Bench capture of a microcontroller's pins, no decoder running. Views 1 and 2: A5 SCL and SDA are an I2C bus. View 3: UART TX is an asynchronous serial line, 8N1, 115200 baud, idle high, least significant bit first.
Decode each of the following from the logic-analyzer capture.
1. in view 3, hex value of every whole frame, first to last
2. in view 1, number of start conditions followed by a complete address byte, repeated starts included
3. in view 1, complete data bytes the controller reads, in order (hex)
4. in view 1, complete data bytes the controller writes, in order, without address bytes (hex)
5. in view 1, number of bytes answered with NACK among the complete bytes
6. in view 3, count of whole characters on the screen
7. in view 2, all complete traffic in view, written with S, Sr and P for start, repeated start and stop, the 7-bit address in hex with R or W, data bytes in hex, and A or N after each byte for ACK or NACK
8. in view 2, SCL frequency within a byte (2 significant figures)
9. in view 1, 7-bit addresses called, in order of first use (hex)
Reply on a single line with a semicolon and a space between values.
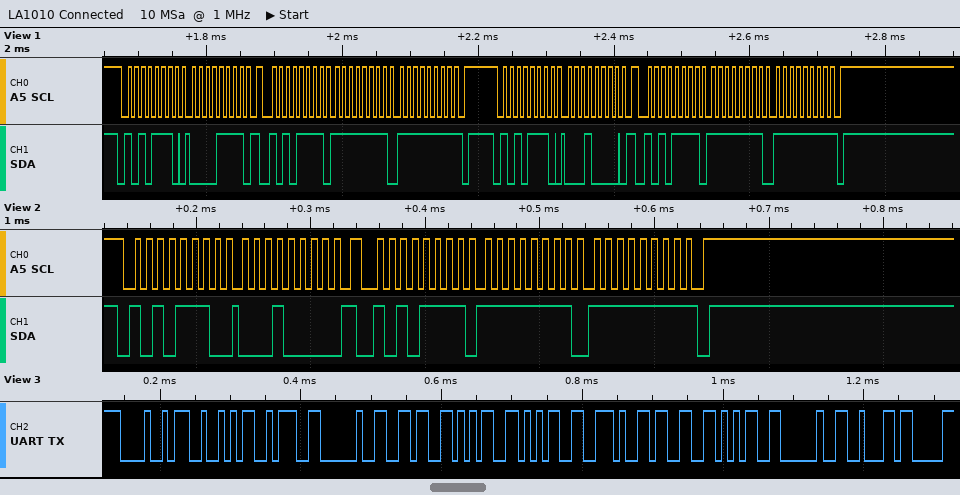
48 52 3A 20 36 35 35 2E 33 35 20 62; 4; FF FF FF FF; 0F 10; 2; 12; S 57W A 10 A Sr 57R A FF A FF N P; 100 kHz; 0x57
